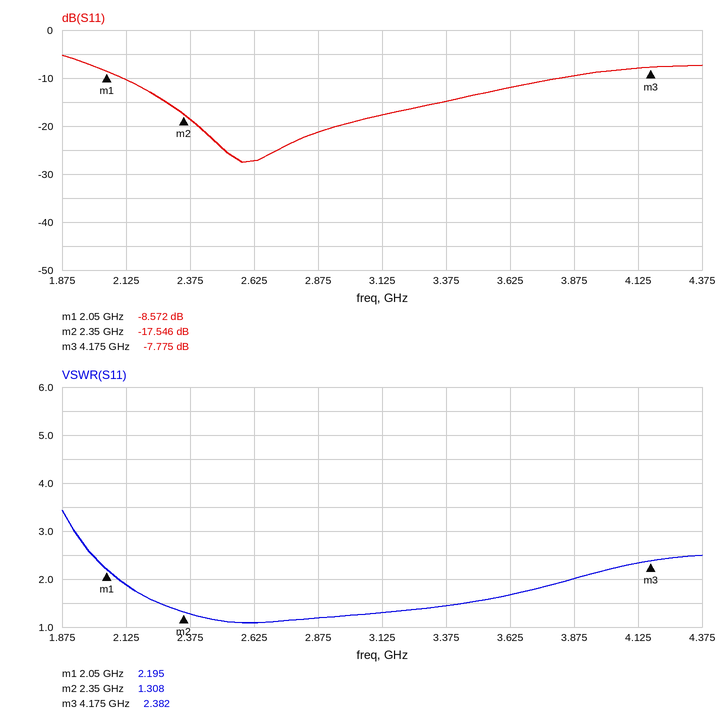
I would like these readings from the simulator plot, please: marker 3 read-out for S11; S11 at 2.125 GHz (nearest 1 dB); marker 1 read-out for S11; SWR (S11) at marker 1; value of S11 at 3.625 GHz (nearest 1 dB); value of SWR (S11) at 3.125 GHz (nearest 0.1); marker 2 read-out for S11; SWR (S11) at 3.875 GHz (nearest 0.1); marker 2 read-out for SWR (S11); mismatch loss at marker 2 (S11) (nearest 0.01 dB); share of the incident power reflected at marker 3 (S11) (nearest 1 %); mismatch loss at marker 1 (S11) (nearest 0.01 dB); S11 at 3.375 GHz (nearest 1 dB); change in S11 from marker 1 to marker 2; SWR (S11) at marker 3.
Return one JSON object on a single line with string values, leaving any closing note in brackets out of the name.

{"marker 3 read-out for S11": "-7.775 dB", "S11 at 2.125 GHz": "-10 dB", "marker 1 read-out for S11": "-8.572 dB", "SWR (S11) at marker 1": "2.195", "value of S11 at 3.625 GHz": "-12 dB", "value of SWR (S11) at 3.125 GHz": "1.3", "marker 2 read-out for S11": "-17.546 dB", "SWR (S11) at 3.875 GHz": "2.0", "marker 2 read-out for SWR": "1.308", "mismatch loss at marker 2 (S11)": "0.08 dB", "share of the incident power reflected at marker 3 (S11)": "17 %", "mismatch loss at marker 1 (S11)": "0.65 dB", "S11 at 3.375 GHz": "-15 dB", "change in S11 from marker 1 to marker 2": "-8.974 dB", "SWR (S11) at marker 3": "2.382"}
